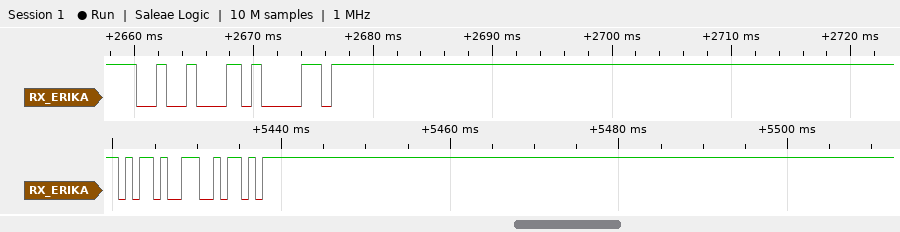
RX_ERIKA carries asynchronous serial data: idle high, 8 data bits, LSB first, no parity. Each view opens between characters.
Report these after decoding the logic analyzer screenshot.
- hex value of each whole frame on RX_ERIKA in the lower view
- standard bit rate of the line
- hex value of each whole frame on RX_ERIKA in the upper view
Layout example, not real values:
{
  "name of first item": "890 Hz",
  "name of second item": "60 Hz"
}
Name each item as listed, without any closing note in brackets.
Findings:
{
  "hex value of each whole frame on RX_ERIKA in the lower view": "2D, 5A",
  "standard bit rate of the line": "1200 baud",
  "hex value of each whole frame on RX_ERIKA in the upper view": "12, 61"
}
